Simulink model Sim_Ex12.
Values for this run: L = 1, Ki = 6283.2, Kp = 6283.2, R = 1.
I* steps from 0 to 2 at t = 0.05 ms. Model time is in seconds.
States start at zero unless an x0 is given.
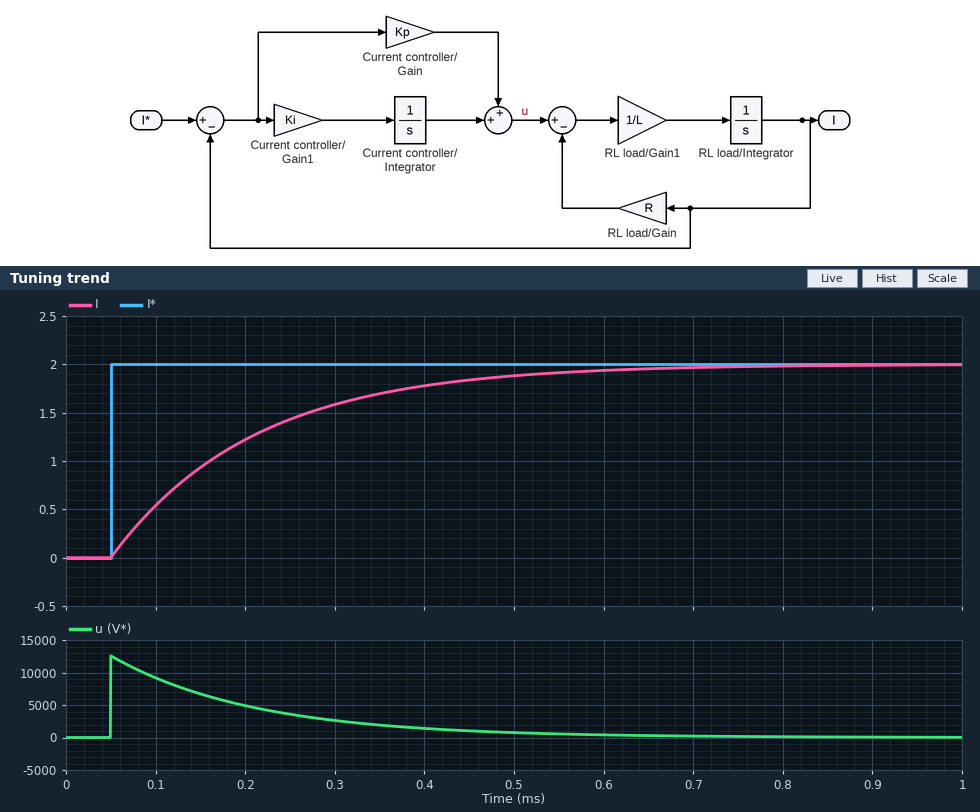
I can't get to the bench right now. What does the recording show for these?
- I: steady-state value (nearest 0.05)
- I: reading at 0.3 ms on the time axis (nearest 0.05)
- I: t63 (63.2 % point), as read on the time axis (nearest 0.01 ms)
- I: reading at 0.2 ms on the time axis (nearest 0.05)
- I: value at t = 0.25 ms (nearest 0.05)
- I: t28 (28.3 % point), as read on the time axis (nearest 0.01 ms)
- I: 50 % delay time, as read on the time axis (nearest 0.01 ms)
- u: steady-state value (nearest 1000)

2.00
1.60
0.21 ms
1.20
1.45
0.10 ms
0.16 ms
0
